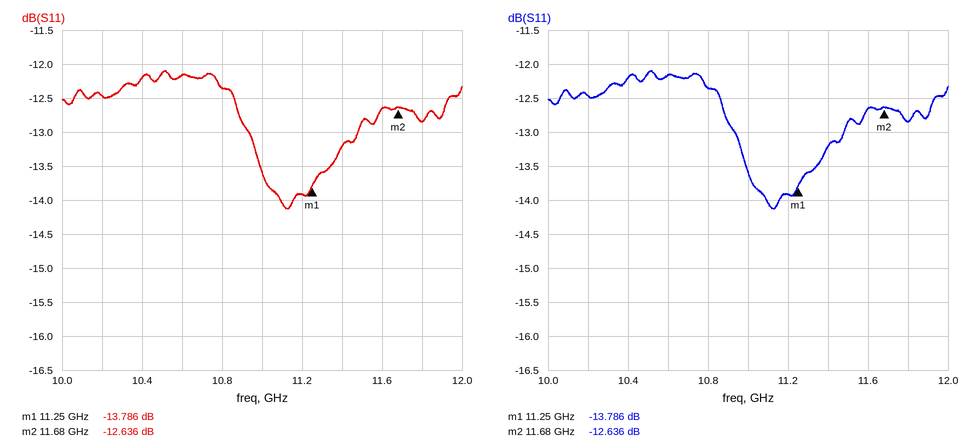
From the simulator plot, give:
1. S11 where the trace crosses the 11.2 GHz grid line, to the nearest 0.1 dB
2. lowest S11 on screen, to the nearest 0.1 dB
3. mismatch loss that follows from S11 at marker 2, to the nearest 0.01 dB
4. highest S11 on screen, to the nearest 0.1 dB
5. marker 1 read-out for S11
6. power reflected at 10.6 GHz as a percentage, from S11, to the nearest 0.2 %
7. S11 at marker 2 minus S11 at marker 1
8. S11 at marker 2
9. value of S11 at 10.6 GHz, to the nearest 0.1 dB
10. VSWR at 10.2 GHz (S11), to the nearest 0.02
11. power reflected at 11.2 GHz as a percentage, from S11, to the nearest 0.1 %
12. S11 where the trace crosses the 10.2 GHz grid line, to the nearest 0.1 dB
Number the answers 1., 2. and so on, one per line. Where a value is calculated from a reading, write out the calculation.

1. -13.9 dB
2. -14.1 dB
3. −10 log10(1 − 10^(-12.636/10)) ≈ 0.24 dB
4. -12.1 dB
5. -13.786 dB
6. 10^(-12.2/10) ≈ 6.0 %
7. -12.636 − (-13.786) = 1.150 dB
8. -12.636 dB
9. -12.2 dB
10. |Γ| = 10^(-12.5/20) = 0.2371; VSWR = (1 + 0.2371)/(1 − 0.2371) ≈ 1.62
11. 10^(-13.9/10) ≈ 4.1 %
12. -12.5 dB
